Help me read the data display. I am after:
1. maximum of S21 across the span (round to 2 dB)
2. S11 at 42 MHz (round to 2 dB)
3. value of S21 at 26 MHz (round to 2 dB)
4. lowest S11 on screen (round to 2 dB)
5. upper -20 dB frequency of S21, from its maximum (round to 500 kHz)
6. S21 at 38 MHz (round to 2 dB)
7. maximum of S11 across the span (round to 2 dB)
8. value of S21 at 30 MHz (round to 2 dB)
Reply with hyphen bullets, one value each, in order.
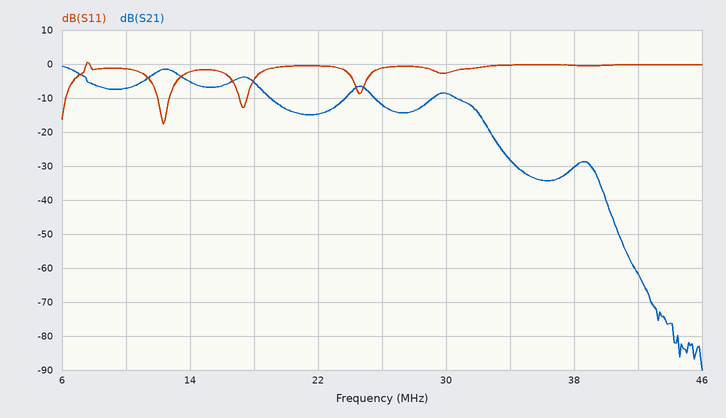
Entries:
- 0 dB
- 0 dB
- -12 dB
- -18 dB
- 33.0 MHz
- -30 dB
- 0 dB
- -8 dB
